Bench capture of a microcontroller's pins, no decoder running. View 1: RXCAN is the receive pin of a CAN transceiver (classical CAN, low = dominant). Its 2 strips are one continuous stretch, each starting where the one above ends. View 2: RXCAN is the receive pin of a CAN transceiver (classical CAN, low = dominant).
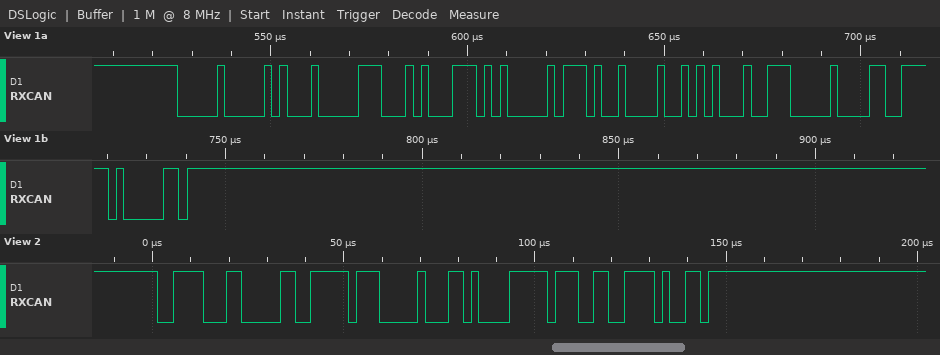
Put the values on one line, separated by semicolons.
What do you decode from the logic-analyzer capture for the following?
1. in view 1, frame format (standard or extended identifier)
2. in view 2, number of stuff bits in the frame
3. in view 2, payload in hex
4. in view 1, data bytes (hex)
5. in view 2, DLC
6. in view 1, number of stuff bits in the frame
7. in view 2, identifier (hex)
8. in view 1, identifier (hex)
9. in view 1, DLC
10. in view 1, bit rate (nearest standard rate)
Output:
standard; 4; FF 00 D0 FF; 31 47 50 3A 42 54 4E 00; 4; 7; 0x3C6; 0x001; 8; 500 kbit/s
